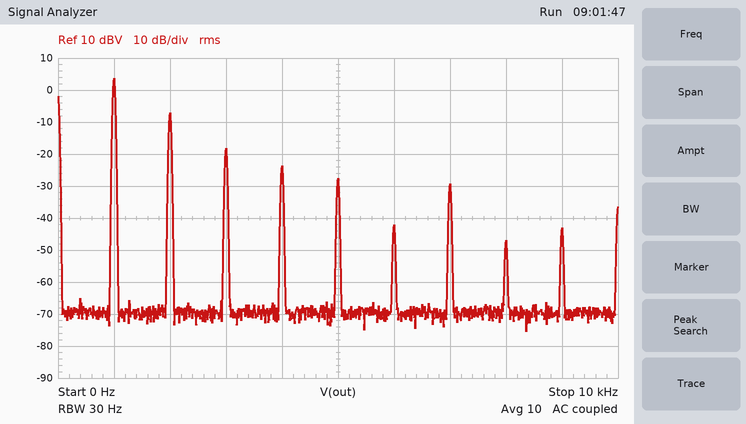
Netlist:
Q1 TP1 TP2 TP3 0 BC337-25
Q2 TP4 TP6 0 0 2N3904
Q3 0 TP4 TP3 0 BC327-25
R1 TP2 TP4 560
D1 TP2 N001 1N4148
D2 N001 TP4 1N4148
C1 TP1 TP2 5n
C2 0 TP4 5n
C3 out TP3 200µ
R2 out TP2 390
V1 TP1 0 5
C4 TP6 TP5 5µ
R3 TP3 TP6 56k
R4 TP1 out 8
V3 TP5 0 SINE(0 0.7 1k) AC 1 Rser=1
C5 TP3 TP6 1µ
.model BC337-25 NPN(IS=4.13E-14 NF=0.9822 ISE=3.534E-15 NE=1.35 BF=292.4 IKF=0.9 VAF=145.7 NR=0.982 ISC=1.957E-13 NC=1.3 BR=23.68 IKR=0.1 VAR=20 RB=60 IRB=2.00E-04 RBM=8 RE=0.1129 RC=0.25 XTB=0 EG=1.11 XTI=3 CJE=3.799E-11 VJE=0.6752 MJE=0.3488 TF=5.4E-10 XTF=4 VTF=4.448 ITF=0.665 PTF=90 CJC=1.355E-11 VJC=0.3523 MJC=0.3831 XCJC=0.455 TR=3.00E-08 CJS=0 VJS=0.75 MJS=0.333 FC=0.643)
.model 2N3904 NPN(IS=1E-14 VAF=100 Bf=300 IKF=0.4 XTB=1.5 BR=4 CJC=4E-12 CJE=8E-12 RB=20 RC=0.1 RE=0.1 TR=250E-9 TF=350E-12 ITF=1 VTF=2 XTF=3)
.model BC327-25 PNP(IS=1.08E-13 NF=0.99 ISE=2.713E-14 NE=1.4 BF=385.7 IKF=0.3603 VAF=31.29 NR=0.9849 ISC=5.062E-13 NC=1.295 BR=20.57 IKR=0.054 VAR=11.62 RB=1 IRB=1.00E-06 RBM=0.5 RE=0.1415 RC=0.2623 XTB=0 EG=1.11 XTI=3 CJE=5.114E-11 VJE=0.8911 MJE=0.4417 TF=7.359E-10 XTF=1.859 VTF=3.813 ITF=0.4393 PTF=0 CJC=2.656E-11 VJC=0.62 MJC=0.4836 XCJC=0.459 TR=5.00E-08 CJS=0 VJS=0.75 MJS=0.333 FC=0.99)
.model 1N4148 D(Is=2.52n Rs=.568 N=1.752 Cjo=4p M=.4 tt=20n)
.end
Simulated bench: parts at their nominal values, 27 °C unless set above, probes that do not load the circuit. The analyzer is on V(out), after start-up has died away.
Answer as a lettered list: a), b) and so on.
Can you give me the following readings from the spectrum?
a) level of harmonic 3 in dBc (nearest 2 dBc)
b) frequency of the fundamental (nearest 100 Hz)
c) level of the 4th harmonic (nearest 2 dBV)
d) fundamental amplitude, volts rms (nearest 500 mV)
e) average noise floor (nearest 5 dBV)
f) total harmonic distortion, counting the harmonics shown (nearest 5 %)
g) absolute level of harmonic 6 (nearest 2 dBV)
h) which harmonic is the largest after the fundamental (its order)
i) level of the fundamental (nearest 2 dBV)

a) -22 dBc
b) 1.0 kHz
c) -24 dBV
d) 1.5 V
e) -70 dBV
f) 30 %
g) -42 dBV
h) 2
i) 4 dBV
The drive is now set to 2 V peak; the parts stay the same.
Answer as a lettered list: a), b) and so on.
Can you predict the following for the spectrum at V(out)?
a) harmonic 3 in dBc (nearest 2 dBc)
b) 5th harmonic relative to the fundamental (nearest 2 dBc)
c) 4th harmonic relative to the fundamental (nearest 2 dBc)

a) -8 dBc
b) -24 dBc
c) -20 dBc
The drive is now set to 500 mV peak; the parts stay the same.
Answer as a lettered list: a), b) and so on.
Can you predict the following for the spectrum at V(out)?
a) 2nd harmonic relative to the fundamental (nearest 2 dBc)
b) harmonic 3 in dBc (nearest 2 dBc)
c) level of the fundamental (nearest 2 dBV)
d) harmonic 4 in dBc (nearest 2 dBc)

a) -22 dBc
b) -24 dBc
c) 4 dBV
d) -32 dBc
